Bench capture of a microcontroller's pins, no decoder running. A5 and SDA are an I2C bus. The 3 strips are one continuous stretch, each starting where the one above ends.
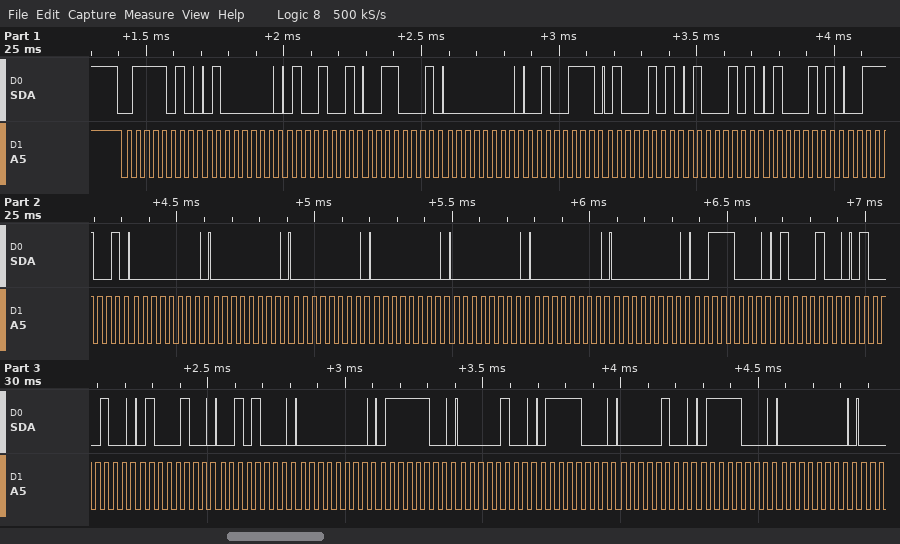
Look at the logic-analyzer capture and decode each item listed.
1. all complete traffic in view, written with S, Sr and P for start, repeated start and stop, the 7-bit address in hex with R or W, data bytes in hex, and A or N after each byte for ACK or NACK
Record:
S 3DW A 40 A 49 A 31 A 00 A 27 A 45 A 45 A 45 A 39 A 00 A 00 A 00 A 00 A 00 A 00 A 00 A 38 A 44 A 44 A 44 A 28 A 00 A 7C A 04 A 78 A 04 A 78 A 00 A
